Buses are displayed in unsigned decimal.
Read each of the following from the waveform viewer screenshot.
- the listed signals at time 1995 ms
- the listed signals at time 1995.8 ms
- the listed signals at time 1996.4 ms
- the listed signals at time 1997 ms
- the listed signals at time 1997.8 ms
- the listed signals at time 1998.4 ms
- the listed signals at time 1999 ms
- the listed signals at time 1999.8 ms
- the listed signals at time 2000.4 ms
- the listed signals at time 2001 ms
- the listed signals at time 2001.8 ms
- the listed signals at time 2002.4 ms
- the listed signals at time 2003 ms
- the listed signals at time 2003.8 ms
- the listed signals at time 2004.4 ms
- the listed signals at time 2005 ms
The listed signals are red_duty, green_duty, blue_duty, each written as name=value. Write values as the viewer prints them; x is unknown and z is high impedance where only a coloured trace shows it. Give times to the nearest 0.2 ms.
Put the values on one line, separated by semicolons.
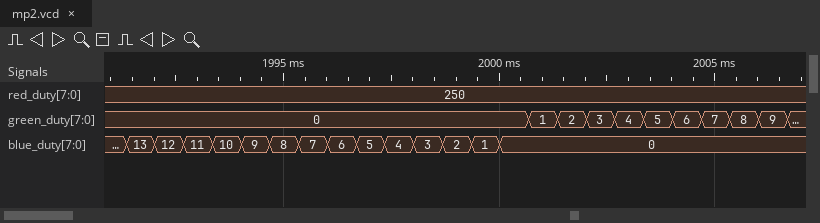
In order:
red_duty=250, green_duty=0, blue_duty=8; red_duty=250, green_duty=0, blue_duty=7; red_duty=250, green_duty=0, blue_duty=6; red_duty=250, green_duty=0, blue_duty=5; red_duty=250, green_duty=0, blue_duty=4; red_duty=250, green_duty=0, blue_duty=3; red_duty=250, green_duty=0, blue_duty=2; red_duty=250, green_duty=0, blue_duty=1; red_duty=250, green_duty=0, blue_duty=0; red_duty=250, green_duty=1, blue_duty=0; red_duty=250, green_duty=2, blue_duty=0; red_duty=250, green_duty=3, blue_duty=0; red_duty=250, green_duty=4, blue_duty=0; red_duty=250, green_duty=5, blue_duty=0; red_duty=250, green_duty=6, blue_duty=0; red_duty=250, green_duty=7, blue_duty=0
